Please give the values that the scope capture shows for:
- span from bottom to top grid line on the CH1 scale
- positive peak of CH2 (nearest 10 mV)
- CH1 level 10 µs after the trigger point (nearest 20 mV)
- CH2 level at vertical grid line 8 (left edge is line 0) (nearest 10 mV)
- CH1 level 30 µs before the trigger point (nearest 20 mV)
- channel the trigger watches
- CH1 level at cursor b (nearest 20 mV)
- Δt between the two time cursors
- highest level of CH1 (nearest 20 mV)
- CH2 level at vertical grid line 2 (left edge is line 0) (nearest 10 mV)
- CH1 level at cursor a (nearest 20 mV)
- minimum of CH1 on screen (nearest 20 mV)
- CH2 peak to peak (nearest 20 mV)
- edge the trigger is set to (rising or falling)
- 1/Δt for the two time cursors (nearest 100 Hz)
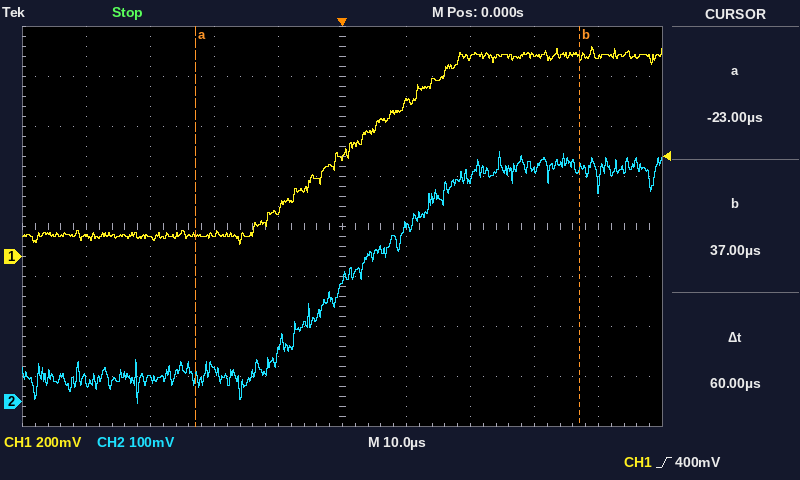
1.6 V
500 mV
620 mV
460 mV
80 mV
CH1
800 mV
60 µs
840 mV
40 mV
80 mV
40 mV
500 mV
rising
16.7 kHz
